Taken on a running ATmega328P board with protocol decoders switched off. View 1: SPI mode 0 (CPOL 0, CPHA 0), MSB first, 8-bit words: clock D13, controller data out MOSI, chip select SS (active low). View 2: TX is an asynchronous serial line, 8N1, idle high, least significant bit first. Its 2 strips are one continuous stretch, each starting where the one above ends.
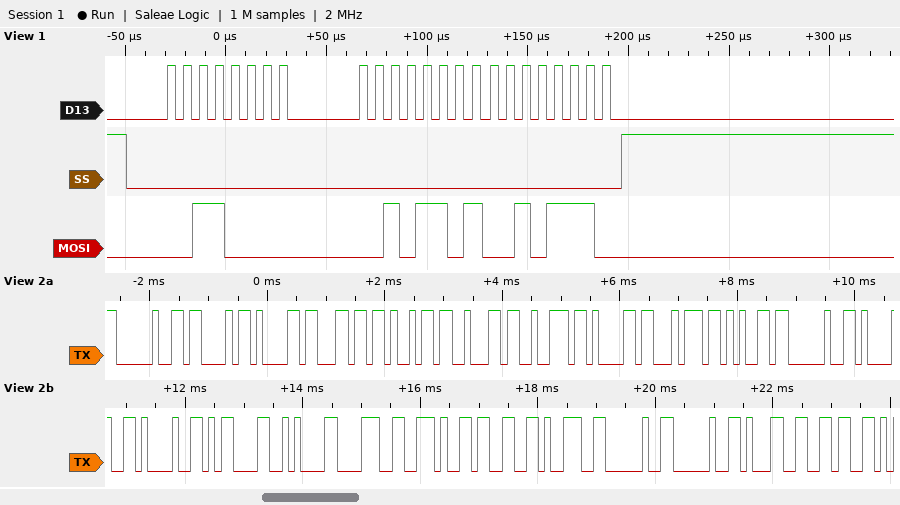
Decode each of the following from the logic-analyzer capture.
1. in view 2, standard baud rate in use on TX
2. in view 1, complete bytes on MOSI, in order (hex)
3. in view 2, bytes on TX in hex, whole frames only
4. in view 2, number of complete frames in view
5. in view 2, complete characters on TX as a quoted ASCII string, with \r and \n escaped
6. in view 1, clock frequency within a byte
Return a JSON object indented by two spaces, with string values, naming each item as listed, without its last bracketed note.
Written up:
{
  "in view 2, standard baud rate in use on TX": "9600 baud",
  "in view 1, complete bytes on MOSI, in order": "30 2D 2E",
  "in view 2, bytes on TX in hex, whole frames only": "20 43 61 6C 69 62 72 61 74 65 20 21 21 0D 0A 38 2E 33 39 20 20 31 36",
  "in view 2, number of complete frames in view": "23",
  "in view 2, complete characters on TX as a quoted ASCII string, with \\r and \\n escaped": "\" Calibrate !!\\r\\n8.39  16\"",
  "in view 1, clock frequency within a byte": "125 kHz"
}
